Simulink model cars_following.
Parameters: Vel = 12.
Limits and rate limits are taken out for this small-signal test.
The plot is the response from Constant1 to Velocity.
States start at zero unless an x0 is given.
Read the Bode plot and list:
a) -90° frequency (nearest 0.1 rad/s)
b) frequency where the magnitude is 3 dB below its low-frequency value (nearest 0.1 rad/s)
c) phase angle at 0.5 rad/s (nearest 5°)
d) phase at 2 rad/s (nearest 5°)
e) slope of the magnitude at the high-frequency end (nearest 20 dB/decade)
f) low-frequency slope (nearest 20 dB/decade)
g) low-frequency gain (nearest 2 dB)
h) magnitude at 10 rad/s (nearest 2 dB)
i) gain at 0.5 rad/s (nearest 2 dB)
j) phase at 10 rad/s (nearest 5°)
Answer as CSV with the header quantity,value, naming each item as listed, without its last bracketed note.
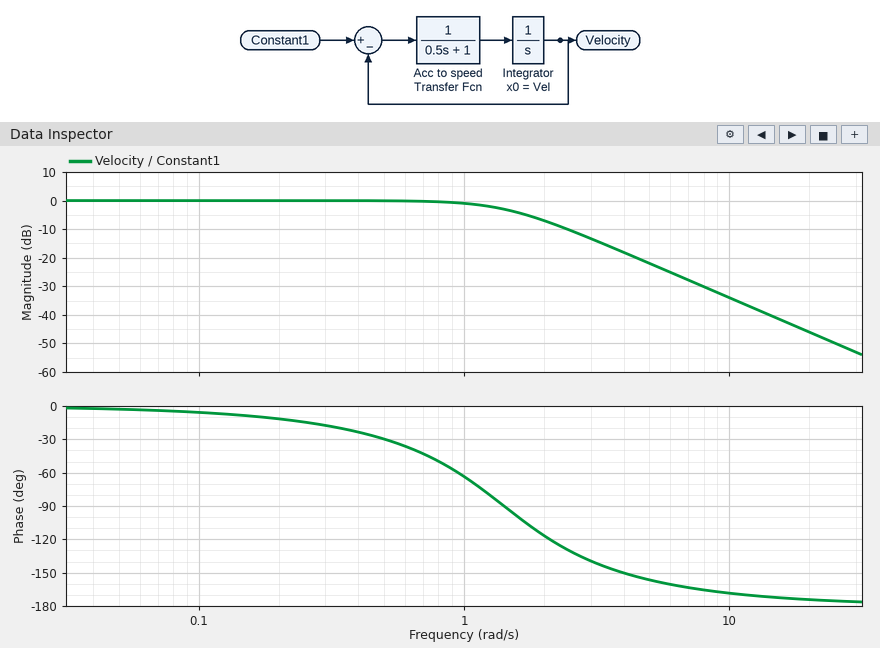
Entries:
quantity,value
-90° frequency,1.4 rad/s
frequency where the magnitude is 3 dB below its low-frequency value,1.4 rad/s
phase angle at 0.5 rad/s,-30°
phase at 2 rad/s,-115°
slope of the magnitude at the high-frequency end,-40 dB/decade
low-frequency slope,0 dB/decade
low-frequency gain,0 dB
magnitude at 10 rad/s,-34 dB
gain at 0.5 rad/s,0 dB
phase at 10 rad/s,-170°
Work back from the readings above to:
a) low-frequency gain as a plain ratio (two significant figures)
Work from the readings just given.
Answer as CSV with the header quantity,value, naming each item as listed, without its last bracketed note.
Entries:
quantity,value
low-frequency gain as a plain ratio,1.0
